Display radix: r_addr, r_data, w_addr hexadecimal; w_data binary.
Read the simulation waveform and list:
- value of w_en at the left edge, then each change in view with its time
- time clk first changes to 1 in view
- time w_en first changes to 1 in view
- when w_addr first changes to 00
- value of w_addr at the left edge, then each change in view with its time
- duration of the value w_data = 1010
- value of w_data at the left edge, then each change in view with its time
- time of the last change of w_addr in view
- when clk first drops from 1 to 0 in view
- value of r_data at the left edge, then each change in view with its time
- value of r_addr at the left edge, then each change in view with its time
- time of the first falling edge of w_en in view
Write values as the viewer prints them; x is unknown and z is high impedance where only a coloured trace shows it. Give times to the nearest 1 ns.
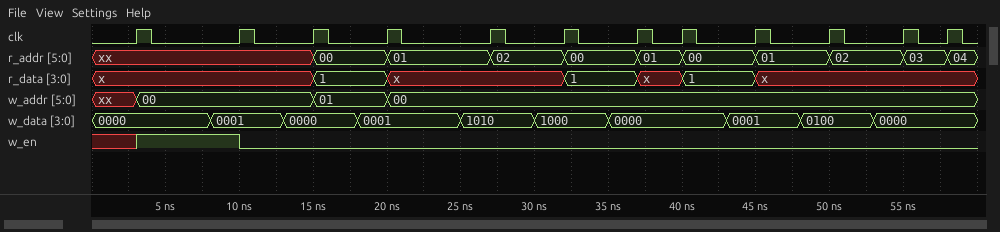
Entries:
x, 1 at 3 ns, 0 at 10 ns
3 ns
3 ns
3 ns
xx, 00 at 3 ns, 01 at 15 ns, 00 at 20 ns
5 ns
0000, 0001 at 8 ns, 0000 at 13 ns, 0001 at 18 ns, 1010 at 25 ns, 1000 at 30 ns, 0000 at 35 ns, 0001 at 43 ns, 0100 at 48 ns, 0000 at 53 ns
20 ns
4 ns
x, 1 at 15 ns, x at 20 ns, 1 at 32 ns, x at 37 ns, 1 at 40 ns, x at 45 ns
xx, 00 at 15 ns, 01 at 20 ns, 02 at 27 ns, 00 at 32 ns, 01 at 37 ns, 00 at 40 ns, 01 at 45 ns, 02 at 50 ns, 03 at 55 ns, 04 at 58 ns
10 ns
